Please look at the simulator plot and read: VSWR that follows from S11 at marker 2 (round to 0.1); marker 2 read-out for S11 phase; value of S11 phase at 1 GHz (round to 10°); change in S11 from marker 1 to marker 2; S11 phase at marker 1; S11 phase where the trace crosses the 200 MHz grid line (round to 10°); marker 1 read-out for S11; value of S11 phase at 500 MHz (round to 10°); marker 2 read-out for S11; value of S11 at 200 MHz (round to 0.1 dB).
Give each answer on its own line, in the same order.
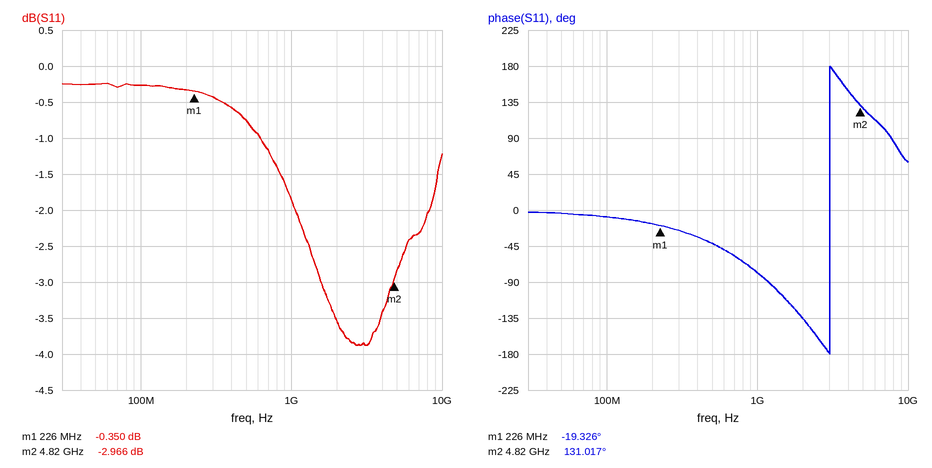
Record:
5.9
131.017°
-80°
-2.616 dB
-19.326°
-20°
-0.350 dB
-40°
-2.966 dB
-0.3 dB
